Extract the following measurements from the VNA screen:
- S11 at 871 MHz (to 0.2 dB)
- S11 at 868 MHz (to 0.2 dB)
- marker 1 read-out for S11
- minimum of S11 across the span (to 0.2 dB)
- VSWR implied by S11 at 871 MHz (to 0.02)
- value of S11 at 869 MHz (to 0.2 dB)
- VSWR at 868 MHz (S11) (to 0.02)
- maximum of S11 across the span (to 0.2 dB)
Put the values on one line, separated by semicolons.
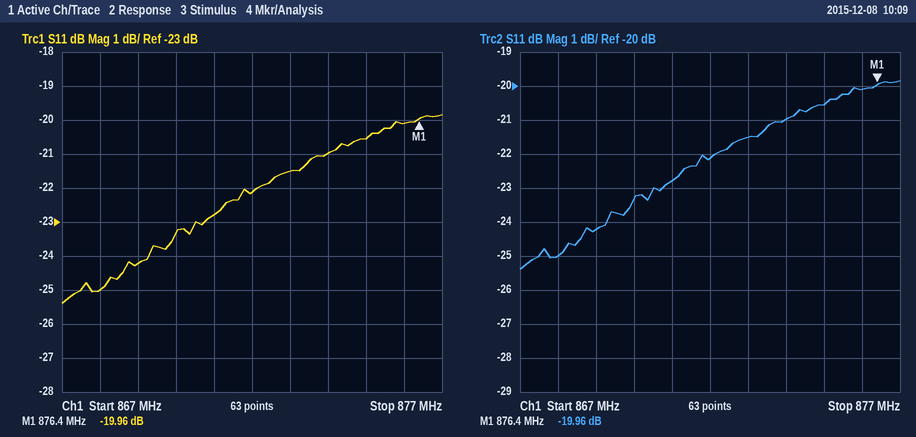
-22.8 dB; -25.0 dB; -19.96 dB; -25.4 dB; 1.16; -24.2 dB; 1.12; -19.8 dB
